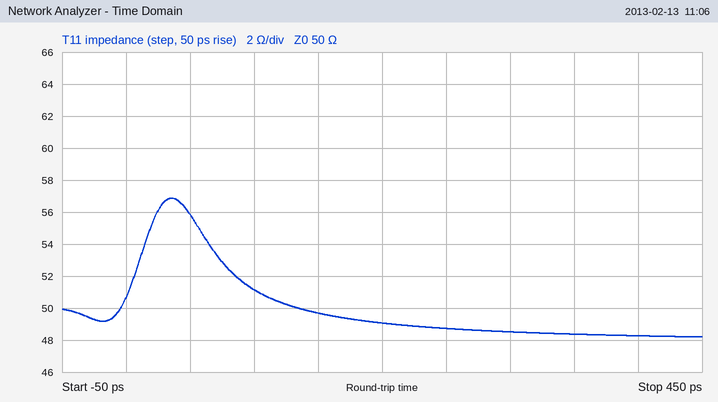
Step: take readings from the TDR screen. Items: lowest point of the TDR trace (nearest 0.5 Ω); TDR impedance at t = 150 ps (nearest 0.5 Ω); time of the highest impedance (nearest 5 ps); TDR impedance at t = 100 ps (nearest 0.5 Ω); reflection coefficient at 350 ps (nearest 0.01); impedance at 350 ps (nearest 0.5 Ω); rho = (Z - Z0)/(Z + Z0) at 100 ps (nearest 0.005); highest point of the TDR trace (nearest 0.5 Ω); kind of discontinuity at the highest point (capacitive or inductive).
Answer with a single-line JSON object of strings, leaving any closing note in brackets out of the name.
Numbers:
{"lowest point of the TDR trace": "48.0 Ω", "TDR impedance at t = 150 ps": "49.5 Ω", "time of the highest impedance": "35 ps", "TDR impedance at t = 100 ps": "51.0 Ω", "reflection coefficient at 350 ps": "-0.02", "impedance at 350 ps": "48.5 Ω", "rho = (Z - Z0)/(Z + Z0) at 100 ps": "+0.010", "highest point of the TDR trace": "57.0 Ω", "kind of discontinuity at the highest point": "inductive"}
